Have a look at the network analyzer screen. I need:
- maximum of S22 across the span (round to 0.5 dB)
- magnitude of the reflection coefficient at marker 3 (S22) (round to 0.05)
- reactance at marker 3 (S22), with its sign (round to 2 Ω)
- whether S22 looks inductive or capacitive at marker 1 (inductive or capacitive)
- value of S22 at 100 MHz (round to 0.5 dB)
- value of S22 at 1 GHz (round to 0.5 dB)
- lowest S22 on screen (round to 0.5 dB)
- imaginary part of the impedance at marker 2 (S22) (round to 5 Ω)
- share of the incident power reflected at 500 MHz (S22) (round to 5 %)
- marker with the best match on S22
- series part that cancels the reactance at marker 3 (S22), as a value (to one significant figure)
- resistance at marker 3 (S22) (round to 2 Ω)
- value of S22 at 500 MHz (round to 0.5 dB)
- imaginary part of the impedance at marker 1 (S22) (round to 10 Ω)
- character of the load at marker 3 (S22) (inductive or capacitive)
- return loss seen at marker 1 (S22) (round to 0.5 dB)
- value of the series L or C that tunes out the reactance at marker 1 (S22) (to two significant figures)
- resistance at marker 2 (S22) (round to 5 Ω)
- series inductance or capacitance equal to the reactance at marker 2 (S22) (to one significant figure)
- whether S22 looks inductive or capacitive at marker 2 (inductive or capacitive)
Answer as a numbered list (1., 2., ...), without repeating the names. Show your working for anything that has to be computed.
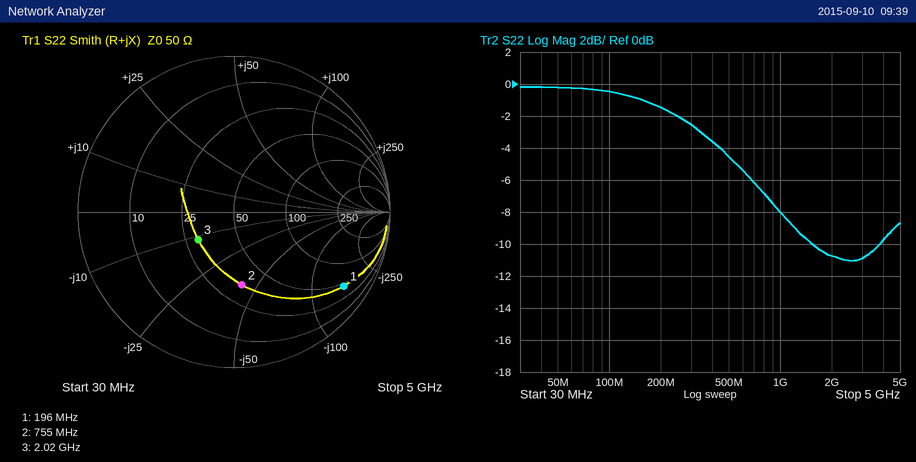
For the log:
1. 0.0 dB
2. 0.30
3. -12 Ω
4. capacitive
5. -0.5 dB
6. -8.0 dB
7. -11.0 dB
8. -40 Ω
9. 10^(-4.5/10) ≈ 35 %
10. marker 3
11. L = 12 Ω/(2π × 2.02 GHz) ≈ 945 pH, so 900 pH to one significant figure
12. 30 Ω
13. -4.5 dB
14. -150 Ω
15. capacitive
16. 1.5 dB
17. L = 150 Ω/(2π × 196 MHz) ≈ 122 nH, so 120 nH to two significant figures
18. 35 Ω
19. C = 1/(2π × 755 MHz × 40 Ω) ≈ 5 pF
20. capacitive
